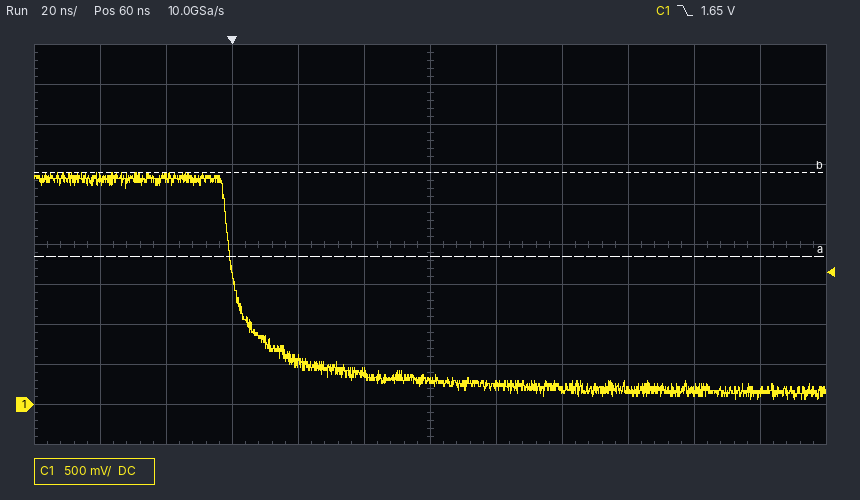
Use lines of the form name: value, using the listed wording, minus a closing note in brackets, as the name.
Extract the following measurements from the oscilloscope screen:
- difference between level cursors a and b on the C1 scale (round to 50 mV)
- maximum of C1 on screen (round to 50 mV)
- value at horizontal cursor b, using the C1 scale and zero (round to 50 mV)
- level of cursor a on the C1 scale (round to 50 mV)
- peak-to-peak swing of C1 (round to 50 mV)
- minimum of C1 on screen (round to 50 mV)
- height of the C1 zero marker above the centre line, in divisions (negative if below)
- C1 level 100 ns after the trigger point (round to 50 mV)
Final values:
difference between level cursors a and b on the C1 scale: 1.05 V
maximum of C1 on screen: 2.90 V
value at horizontal cursor b, using the C1 scale and zero: 2.90 V
level of cursor a on the C1 scale: 1.85 V
peak-to-peak swing of C1: 2.85 V
minimum of C1 on screen: 50 mV
height of the C1 zero marker above the centre line, in divisions: -4.0 div
C1 level 100 ns after the trigger point: 200 mV
